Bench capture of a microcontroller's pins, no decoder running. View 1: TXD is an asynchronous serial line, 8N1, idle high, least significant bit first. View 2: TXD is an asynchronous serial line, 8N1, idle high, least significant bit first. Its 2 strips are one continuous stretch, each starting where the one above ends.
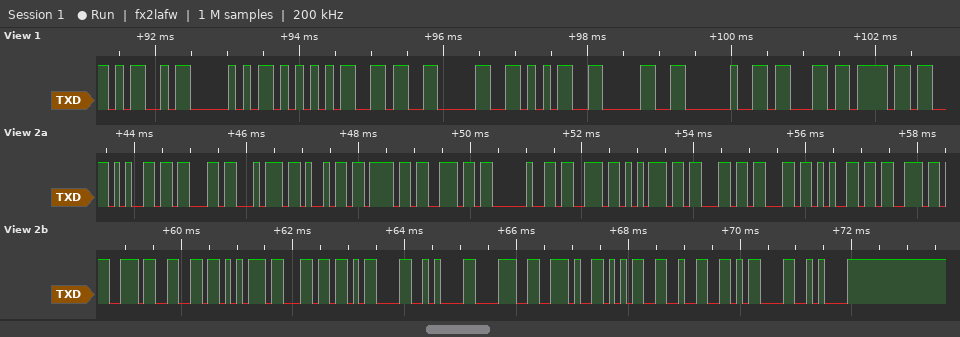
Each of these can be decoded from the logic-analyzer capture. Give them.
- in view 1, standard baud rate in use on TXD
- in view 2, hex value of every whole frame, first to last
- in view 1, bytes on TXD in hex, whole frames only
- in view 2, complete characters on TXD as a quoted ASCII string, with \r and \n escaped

9600 baud
0x65 0x63 0x74 0x69 0x6F 0x6E 0x20 0x73 0x75 0x63 0x63 0x65 0x73 0x73 0x66 0x75 0x6C 0x0D 0x0A 0x38 0x2E 0x35 0x32 0x0D 0x0A
0x4D 0x50 0x55 0x36 0x30 0x35 0x30 0x20 0x63 0x6F
"ection successful\r\n8.52\r\n"
